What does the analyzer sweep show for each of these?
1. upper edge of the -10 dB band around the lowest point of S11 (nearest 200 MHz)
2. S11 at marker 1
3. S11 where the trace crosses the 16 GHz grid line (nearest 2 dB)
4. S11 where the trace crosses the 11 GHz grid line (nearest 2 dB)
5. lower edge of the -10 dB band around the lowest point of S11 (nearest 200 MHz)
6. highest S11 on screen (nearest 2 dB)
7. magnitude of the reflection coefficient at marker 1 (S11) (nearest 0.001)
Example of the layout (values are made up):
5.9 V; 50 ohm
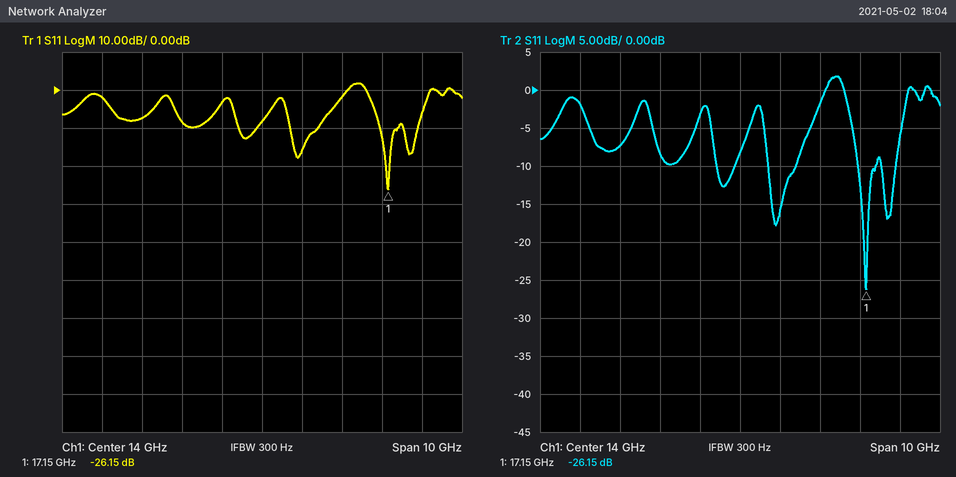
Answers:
17.4 GHz; -26.15 dB; -2 dB; -8 dB; 17.0 GHz; 2 dB; 0.049
